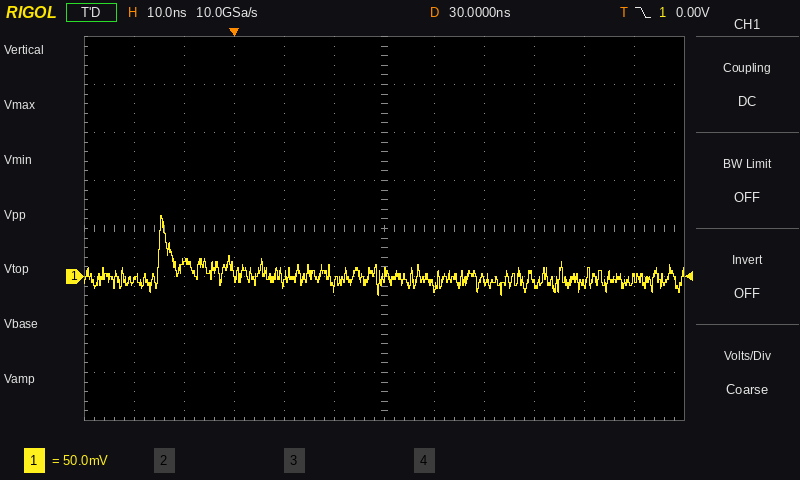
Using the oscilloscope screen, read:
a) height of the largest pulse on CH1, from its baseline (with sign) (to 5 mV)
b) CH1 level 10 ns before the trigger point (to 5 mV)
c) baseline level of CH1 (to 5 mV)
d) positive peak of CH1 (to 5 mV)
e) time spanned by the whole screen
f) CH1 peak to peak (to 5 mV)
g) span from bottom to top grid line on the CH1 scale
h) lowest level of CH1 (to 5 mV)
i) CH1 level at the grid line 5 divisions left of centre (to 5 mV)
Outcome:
+65 mV
15 mV
0 mV
65 mV
120 ns
85 mV
400 mV
-20 mV
-5 mV
